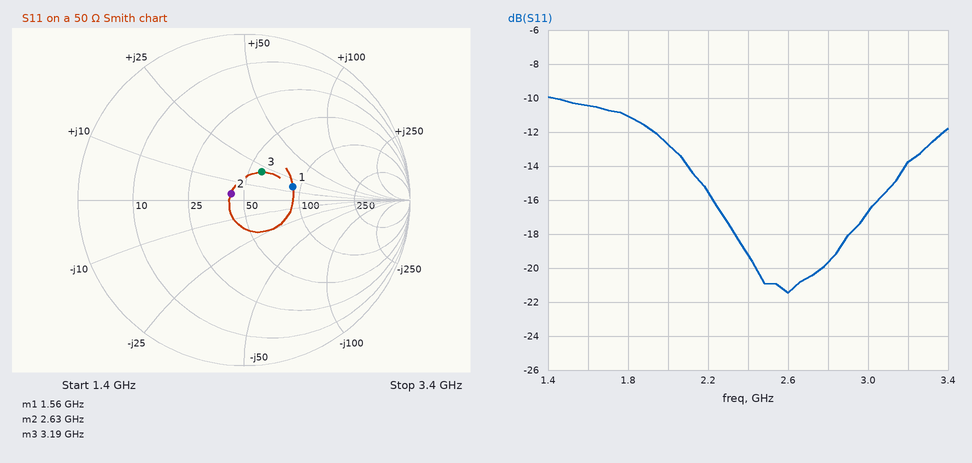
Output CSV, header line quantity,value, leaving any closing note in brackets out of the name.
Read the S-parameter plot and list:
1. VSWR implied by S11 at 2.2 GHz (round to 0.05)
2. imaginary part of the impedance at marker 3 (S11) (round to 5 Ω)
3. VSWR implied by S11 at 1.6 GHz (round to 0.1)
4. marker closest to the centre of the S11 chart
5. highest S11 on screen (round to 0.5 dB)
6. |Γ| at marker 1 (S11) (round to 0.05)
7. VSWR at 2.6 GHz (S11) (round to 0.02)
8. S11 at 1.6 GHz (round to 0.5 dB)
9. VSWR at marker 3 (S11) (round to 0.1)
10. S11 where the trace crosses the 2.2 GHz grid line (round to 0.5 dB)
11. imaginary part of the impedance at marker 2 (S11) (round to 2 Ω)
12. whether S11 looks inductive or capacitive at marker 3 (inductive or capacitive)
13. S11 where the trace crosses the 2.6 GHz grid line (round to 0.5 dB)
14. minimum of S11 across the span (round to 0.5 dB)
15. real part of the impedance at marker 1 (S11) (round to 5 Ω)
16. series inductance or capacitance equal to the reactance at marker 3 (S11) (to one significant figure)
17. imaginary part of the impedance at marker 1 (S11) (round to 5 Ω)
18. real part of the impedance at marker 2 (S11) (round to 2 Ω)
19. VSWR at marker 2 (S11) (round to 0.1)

quantity,value
VSWR implied by S11 at 2.2 GHz,1.40
imaginary part of the impedance at marker 3 (S11),+20 Ω
VSWR implied by S11 at 1.6 GHz,1.9
marker closest to the centre of the S11 chart,marker 2
highest S11 on screen,-10.0 dB
|Γ| at marker 1 (S11),0.30
VSWR at 2.6 GHz (S11),1.18
S11 at 1.6 GHz,-10.5 dB
VSWR at marker 3 (S11),1.5
S11 where the trace crosses the 2.2 GHz grid line,-15.5 dB
imaginary part of the impedance at marker 2 (S11),+4 Ω
whether S11 looks inductive or capacitive at marker 3,inductive
S11 where the trace crosses the 2.6 GHz grid line,-21.5 dB
minimum of S11 across the span,-21.5 dB
real part of the impedance at marker 1 (S11),90 Ω
series inductance or capacitance equal to the reactance at marker 3 (S11),1 nH
imaginary part of the impedance at marker 1 (S11),+15 Ω
real part of the impedance at marker 2 (S11),42 Ω
VSWR at marker 2 (S11),1.2
